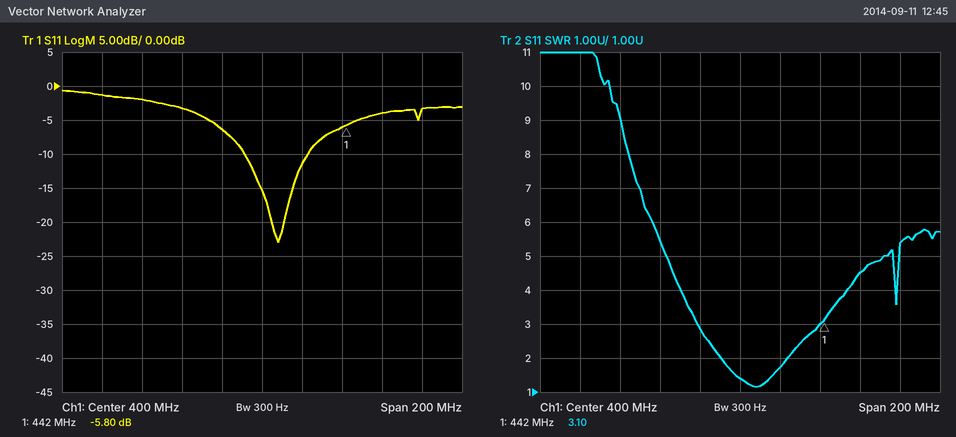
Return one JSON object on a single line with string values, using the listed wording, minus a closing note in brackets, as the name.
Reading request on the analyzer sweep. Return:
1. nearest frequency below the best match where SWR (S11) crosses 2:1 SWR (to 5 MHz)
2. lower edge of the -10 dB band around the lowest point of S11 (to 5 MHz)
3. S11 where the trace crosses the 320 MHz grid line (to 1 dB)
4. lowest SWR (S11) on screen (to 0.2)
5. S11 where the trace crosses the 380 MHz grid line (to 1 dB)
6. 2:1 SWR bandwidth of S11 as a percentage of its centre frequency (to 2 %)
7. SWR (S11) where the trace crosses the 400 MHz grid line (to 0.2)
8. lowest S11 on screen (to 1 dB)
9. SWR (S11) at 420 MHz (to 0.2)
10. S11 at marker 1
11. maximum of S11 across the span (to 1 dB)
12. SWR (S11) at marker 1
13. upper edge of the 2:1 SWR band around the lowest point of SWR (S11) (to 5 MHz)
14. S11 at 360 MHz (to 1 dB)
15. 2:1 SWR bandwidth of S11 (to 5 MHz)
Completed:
{"nearest frequency below the best match where SWR (S11) crosses 2:1 SWR": "390 MHz", "lower edge of the -10 dB band around the lowest point of S11": "390 MHz", "S11 where the trace crosses the 320 MHz grid line": "-1 dB", "lowest SWR (S11) on screen": "1.2", "S11 where the trace crosses the 380 MHz grid line": "-6 dB", "2:1 SWR bandwidth of S11 as a percentage of its centre frequency": "8 %", "SWR (S11) where the trace crosses the 400 MHz grid line": "1.4", "lowest S11 on screen": "-23 dB", "SWR (S11) at 420 MHz": "1.8", "S11 at marker 1": "-5.80 dB", "maximum of S11 across the span": "-1 dB", "SWR (S11) at marker 1": "3.10", "upper edge of the 2:1 SWR band around the lowest point of SWR (S11)": "425 MHz", "S11 at 360 MHz": "-3 dB", "2:1 SWR bandwidth of S11": "35 MHz"}
